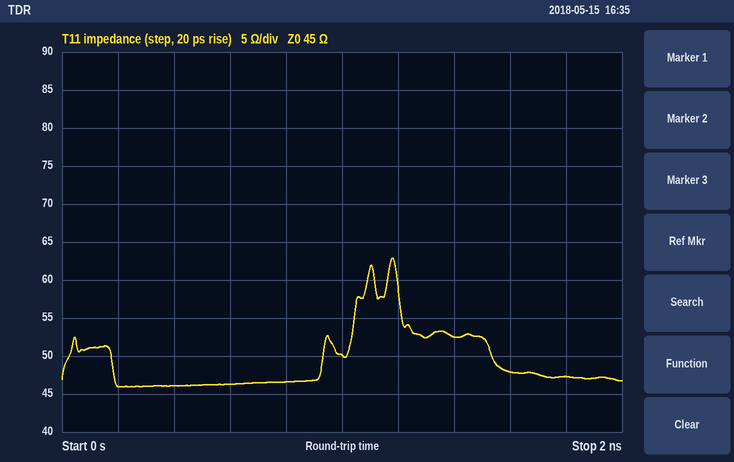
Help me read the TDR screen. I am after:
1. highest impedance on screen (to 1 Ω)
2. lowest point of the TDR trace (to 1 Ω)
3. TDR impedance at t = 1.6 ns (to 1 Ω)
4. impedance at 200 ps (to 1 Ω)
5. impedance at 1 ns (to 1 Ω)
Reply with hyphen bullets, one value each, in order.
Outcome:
- 63 Ω
- 46 Ω
- 48 Ω
- 46 Ω
- 50 Ω
